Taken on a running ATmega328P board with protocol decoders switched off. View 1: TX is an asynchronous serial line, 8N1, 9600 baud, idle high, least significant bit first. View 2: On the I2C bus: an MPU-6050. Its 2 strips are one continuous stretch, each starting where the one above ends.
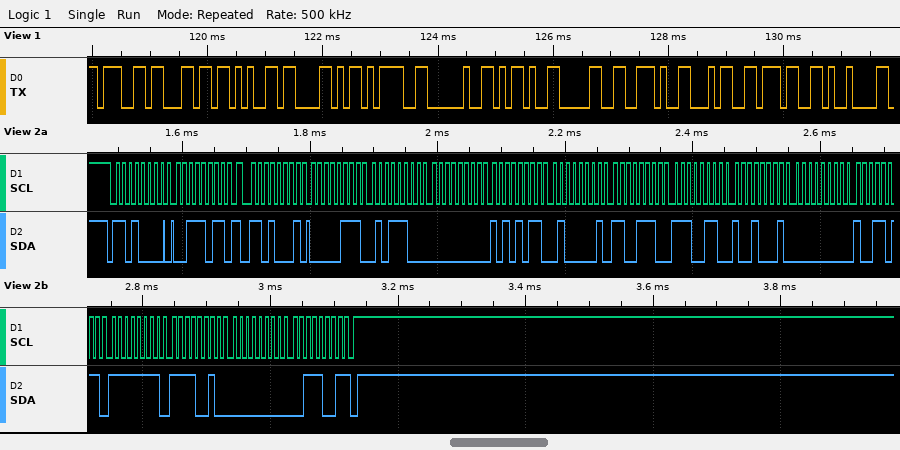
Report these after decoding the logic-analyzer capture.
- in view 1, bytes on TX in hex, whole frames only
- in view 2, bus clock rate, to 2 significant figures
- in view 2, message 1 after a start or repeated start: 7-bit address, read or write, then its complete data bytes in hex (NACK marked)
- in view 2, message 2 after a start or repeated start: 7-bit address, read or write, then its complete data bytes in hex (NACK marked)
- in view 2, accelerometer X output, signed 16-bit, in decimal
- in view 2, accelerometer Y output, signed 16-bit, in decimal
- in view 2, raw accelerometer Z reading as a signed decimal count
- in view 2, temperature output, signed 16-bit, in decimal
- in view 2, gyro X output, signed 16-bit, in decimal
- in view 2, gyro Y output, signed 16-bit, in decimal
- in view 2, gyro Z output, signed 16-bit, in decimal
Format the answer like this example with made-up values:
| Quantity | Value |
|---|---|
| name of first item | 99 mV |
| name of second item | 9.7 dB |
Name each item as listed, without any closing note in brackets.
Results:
| Quantity | Value |
|---|---|
| in view 1, bytes on TX in hex, whole frames only | 0x67 0x6C 0x65 0x58 0x3D 0x20 0x2D 0x30 0x2E 0x34 0x37 0x09 |
| in view 2, bus clock rate, to 2 significant figures | 100 kHz |
| in view 2, message 1 after a start or repeated start: 7-bit address, read or write, then its complete data bytes in hex | 0x68 write: 3B |
| in view 2, message 2 after a start or repeated start: 7-bit address, read or write, then its complete data bytes in hex | 0x68 read: 07 5C 00 AB 41 CE E6 91 00 9B FF F2 00 39 NACK |
| in view 2, accelerometer X output, signed 16-bit, in decimal | 1884 |
| in view 2, accelerometer Y output, signed 16-bit, in decimal | 171 |
| in view 2, raw accelerometer Z reading as a signed decimal count | 16846 |
| in view 2, temperature output, signed 16-bit, in decimal | -6511 |
| in view 2, gyro X output, signed 16-bit, in decimal | 155 |
| in view 2, gyro Y output, signed 16-bit, in decimal | -14 |
| in view 2, gyro Z output, signed 16-bit, in decimal | 57 |
